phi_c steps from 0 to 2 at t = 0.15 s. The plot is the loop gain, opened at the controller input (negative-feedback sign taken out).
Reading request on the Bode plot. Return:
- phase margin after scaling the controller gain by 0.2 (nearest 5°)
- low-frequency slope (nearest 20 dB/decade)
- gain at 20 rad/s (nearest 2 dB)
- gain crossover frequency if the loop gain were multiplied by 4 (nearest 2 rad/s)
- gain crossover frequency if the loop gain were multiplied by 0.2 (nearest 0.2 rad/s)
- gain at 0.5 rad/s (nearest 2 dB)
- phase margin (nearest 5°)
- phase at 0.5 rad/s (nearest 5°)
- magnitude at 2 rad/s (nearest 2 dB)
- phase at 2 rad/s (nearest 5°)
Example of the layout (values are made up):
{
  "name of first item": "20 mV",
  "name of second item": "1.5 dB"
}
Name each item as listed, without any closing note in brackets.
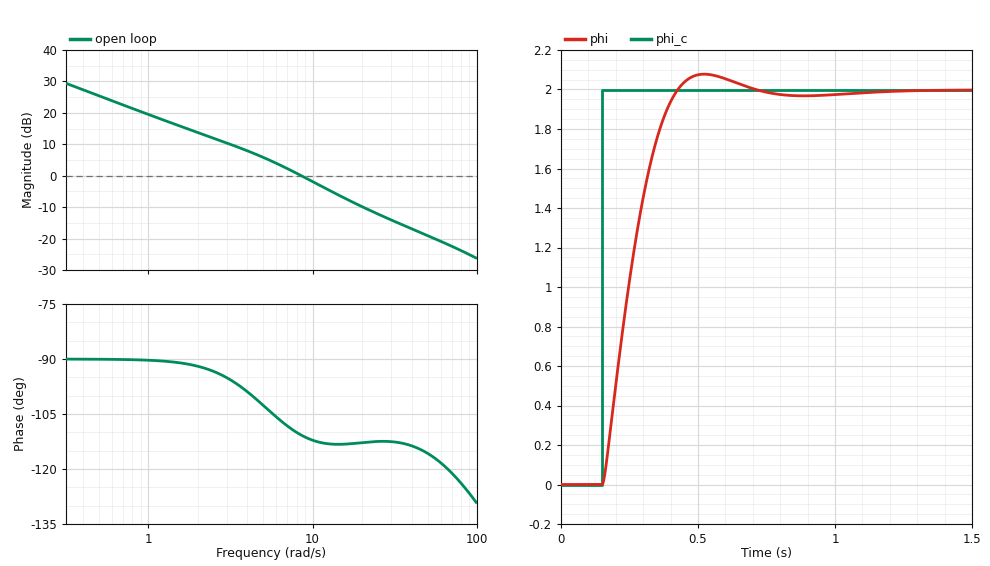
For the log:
{
  "phase margin after scaling the controller gain by 0.2": "90°",
  "low-frequency slope": "-20 dB/decade",
  "gain at 20 rad/s": "-10 dB",
  "gain crossover frequency if the loop gain were multiplied by 4": "24 rad/s",
  "gain crossover frequency if the loop gain were multiplied by 0.2": "2.0 rad/s",
  "gain at 0.5 rad/s": "26 dB",
  "phase margin": "70°",
  "phase at 0.5 rad/s": "-90°",
  "magnitude at 2 rad/s": "14 dB",
  "phase at 2 rad/s": "-90°"
}
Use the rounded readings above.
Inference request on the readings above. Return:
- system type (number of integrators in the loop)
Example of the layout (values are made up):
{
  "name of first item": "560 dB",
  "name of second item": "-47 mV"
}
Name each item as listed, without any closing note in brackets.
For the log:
{
  "system type": "1"
}
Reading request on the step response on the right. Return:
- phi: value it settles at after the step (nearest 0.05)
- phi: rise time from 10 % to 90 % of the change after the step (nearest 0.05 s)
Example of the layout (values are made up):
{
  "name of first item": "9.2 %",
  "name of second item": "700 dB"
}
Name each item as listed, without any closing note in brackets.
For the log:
{
  "phi: value it settles at after the step": "2.00",
  "phi: rise time from 10 % to 90 % of the change after the step": "0.20 s"
}
